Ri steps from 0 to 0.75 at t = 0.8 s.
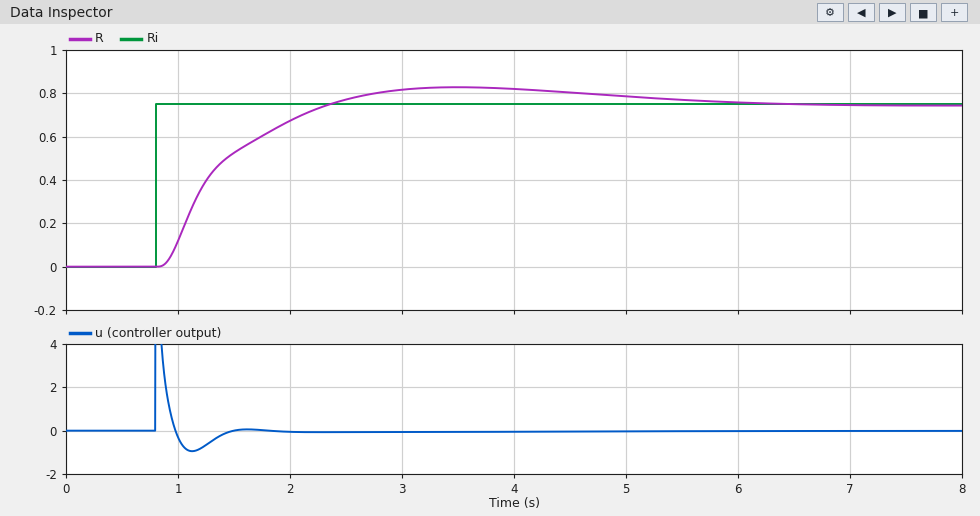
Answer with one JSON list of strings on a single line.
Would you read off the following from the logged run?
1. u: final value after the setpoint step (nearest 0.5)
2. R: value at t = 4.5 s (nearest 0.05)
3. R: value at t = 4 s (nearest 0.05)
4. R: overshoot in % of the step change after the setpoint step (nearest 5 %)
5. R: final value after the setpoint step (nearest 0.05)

["0.0", "0.80", "0.80", "10 %", "0.75"]
